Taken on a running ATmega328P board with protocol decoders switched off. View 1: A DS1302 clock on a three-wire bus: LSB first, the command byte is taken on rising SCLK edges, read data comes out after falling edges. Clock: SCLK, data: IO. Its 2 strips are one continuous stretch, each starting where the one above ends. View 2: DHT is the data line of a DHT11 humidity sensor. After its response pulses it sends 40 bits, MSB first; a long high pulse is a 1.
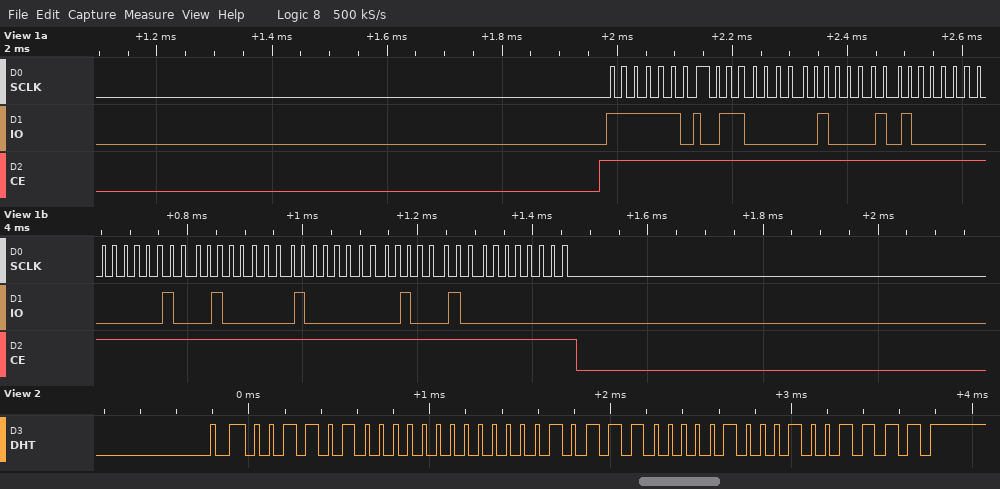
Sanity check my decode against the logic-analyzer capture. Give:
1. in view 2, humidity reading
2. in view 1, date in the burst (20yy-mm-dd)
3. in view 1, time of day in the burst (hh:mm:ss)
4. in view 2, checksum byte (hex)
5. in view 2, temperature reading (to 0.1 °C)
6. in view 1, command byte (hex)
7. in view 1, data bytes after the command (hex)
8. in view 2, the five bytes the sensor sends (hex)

52 %
2022-02-20
01:42:06
0x4F
23.4 °C
0xBF
06 42 01 20 02 01 22 00
34 00 17 04 4F
